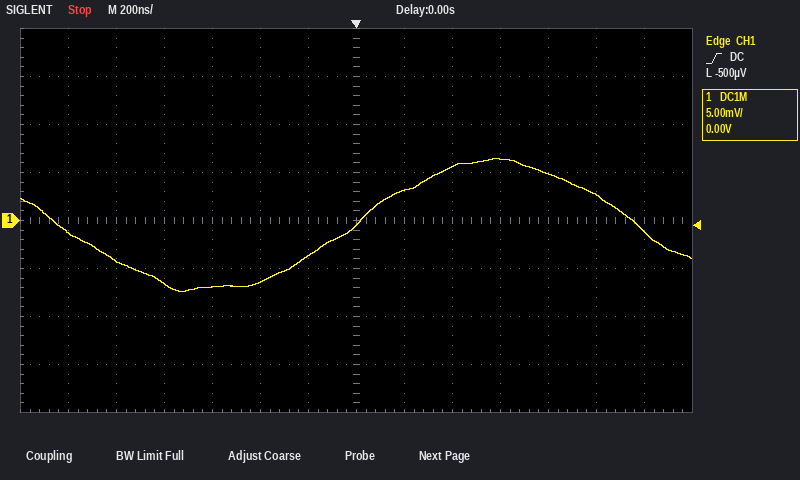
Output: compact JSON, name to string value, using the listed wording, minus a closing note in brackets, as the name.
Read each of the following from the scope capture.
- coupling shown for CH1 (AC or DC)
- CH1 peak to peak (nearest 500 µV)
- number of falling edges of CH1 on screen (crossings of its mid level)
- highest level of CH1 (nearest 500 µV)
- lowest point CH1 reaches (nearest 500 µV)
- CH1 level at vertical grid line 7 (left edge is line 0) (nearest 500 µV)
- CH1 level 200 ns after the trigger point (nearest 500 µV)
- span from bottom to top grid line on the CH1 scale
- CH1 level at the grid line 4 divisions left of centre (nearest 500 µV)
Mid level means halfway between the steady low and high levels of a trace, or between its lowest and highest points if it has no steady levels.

{"coupling shown for CH1": "DC", "CH1 peak to peak": "14.0 mV", "number of falling edges of CH1 on screen": "2", "highest level of CH1": "6.5 mV", "lowest point CH1 reaches": "-7.5 mV", "CH1 level at vertical grid line 7 (left edge is line 0)": "-500 µV", "CH1 level 200 ns after the trigger point": "3.0 mV", "span from bottom to top grid line on the CH1 scale": "40 mV", "CH1 level at the grid line 4 divisions left of centre": "-6.5 mV"}
